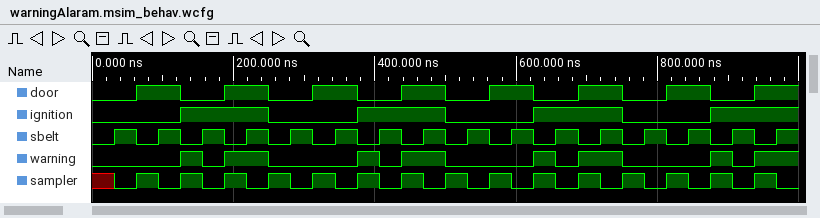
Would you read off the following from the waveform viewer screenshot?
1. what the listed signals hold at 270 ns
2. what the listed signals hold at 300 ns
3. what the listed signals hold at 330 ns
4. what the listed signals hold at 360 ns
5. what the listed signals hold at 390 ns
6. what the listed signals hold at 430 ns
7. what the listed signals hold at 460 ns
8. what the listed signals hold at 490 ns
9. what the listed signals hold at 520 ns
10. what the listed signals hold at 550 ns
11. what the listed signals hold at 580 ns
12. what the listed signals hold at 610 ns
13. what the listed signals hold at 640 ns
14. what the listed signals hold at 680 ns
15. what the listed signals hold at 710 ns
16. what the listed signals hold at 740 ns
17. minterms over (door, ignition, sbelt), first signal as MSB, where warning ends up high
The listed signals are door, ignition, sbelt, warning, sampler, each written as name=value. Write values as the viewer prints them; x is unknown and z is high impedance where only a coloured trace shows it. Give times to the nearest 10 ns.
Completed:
door=0, ignition=0, sbelt=0, warning=0, sampler=1
door=0, ignition=0, sbelt=1, warning=0, sampler=0
door=1, ignition=0, sbelt=0, warning=0, sampler=1
door=1, ignition=0, sbelt=1, warning=0, sampler=0
door=0, ignition=1, sbelt=0, warning=1, sampler=1
door=0, ignition=1, sbelt=1, warning=0, sampler=0
door=1, ignition=1, sbelt=0, warning=1, sampler=1
door=1, ignition=1, sbelt=1, warning=1, sampler=0
door=0, ignition=0, sbelt=0, warning=0, sampler=1
door=0, ignition=0, sbelt=1, warning=0, sampler=0
door=1, ignition=0, sbelt=0, warning=0, sampler=1
door=1, ignition=0, sbelt=1, warning=0, sampler=0
door=0, ignition=1, sbelt=0, warning=1, sampler=1
door=0, ignition=1, sbelt=1, warning=0, sampler=0
door=1, ignition=1, sbelt=0, warning=1, sampler=1
door=1, ignition=1, sbelt=1, warning=1, sampler=0
2, 6, 7
